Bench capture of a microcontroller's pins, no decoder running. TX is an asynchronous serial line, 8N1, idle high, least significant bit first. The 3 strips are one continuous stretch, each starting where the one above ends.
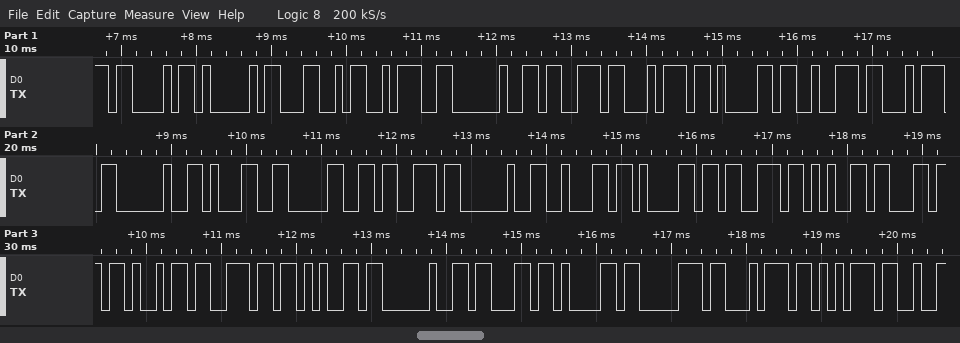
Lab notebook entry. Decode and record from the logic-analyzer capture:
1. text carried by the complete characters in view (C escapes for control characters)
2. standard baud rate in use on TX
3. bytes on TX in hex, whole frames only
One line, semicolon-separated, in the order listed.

"CAL: start 10s baseline captu"; 9600 baud; 43 41 4C 3A 20 73 74 61 72 74 20 31 30 73 20 62 61 73 65 6C 69 6E 65 20 63 61 70 74 75
